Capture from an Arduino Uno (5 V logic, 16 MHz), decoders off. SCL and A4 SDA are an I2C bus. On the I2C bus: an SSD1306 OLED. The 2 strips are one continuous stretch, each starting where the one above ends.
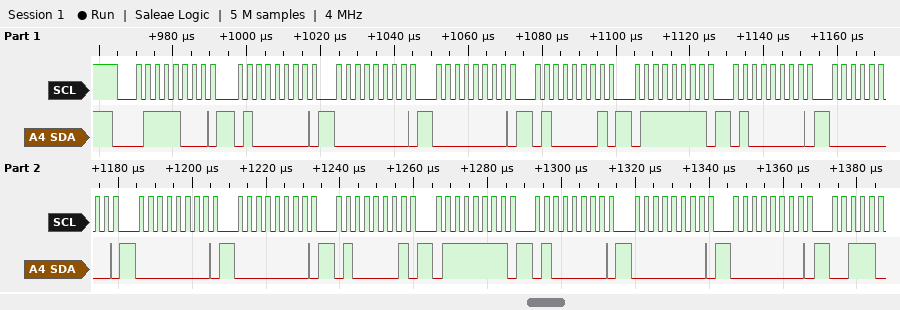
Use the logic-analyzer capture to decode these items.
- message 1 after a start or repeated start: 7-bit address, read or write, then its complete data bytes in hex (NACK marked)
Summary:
0x3C write: 40 00 00 41 7F 40 00 00 00 41 7F 40 00 00
